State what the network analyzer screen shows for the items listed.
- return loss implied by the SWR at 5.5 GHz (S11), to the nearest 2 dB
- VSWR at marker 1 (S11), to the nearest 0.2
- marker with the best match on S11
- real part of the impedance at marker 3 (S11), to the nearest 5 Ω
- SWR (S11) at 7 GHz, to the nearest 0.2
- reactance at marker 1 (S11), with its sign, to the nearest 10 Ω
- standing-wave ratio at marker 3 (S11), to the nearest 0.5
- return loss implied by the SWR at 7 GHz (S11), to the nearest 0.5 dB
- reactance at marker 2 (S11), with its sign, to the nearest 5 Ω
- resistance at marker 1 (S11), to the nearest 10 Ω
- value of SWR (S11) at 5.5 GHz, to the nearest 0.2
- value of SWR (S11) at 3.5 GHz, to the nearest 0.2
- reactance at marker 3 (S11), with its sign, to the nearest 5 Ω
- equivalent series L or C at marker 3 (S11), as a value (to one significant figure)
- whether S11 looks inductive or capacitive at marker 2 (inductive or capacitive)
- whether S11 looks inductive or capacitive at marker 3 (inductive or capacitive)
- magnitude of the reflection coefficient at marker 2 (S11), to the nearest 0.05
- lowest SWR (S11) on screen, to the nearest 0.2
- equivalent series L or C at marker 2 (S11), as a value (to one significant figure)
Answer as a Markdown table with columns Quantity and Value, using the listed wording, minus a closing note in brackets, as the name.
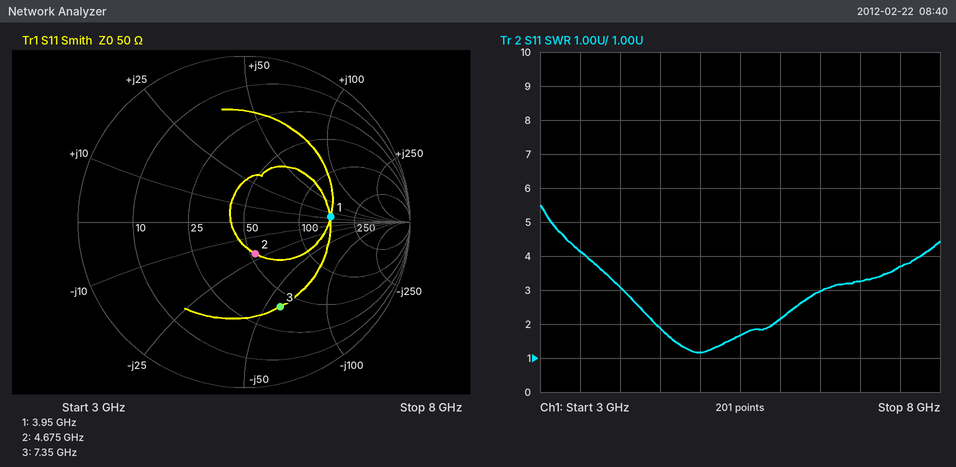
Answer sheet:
| Quantity | Value |
|---|---|
| return loss implied by the SWR at 5.5 GHz (S11), to the nearest 2 dB | 12 dB |
| VSWR at marker 1 (S11), to the nearest 0.2 | 3.2 |
| marker with the best match on S11 | marker 2 |
| real part of the impedance at marker 3 (S11), to the nearest 5 Ω | 40 Ω |
| SWR (S11) at 7 GHz, to the nearest 0.2 | 3.2 |
| reactance at marker 1 (S11), with its sign, to the nearest 10 Ω | +10 Ω |
| standing-wave ratio at marker 3 (S11), to the nearest 0.5 | 3.5 |
| return loss implied by the SWR at 7 GHz (S11), to the nearest 0.5 dB | 5.5 dB |
| reactance at marker 2 (S11), with its sign, to the nearest 5 Ω | -20 Ω |
| resistance at marker 1 (S11), to the nearest 10 Ω | 160 Ω |
| value of SWR (S11) at 5.5 GHz, to the nearest 0.2 | 1.6 |
| value of SWR (S11) at 3.5 GHz, to the nearest 0.2 | 4.2 |
| reactance at marker 3 (S11), with its sign, to the nearest 5 Ω | -60 Ω |
| equivalent series L or C at marker 3 (S11), as a value | 400 fF |
| whether S11 looks inductive or capacitive at marker 2 | capacitive |
| whether S11 looks inductive or capacitive at marker 3 | capacitive |
| magnitude of the reflection coefficient at marker 2 (S11), to the nearest 0.05 | 0.20 |
| lowest SWR (S11) on screen, to the nearest 0.2 | 1.2 |
| equivalent series L or C at marker 2 (S11), as a value | 2 pF |
